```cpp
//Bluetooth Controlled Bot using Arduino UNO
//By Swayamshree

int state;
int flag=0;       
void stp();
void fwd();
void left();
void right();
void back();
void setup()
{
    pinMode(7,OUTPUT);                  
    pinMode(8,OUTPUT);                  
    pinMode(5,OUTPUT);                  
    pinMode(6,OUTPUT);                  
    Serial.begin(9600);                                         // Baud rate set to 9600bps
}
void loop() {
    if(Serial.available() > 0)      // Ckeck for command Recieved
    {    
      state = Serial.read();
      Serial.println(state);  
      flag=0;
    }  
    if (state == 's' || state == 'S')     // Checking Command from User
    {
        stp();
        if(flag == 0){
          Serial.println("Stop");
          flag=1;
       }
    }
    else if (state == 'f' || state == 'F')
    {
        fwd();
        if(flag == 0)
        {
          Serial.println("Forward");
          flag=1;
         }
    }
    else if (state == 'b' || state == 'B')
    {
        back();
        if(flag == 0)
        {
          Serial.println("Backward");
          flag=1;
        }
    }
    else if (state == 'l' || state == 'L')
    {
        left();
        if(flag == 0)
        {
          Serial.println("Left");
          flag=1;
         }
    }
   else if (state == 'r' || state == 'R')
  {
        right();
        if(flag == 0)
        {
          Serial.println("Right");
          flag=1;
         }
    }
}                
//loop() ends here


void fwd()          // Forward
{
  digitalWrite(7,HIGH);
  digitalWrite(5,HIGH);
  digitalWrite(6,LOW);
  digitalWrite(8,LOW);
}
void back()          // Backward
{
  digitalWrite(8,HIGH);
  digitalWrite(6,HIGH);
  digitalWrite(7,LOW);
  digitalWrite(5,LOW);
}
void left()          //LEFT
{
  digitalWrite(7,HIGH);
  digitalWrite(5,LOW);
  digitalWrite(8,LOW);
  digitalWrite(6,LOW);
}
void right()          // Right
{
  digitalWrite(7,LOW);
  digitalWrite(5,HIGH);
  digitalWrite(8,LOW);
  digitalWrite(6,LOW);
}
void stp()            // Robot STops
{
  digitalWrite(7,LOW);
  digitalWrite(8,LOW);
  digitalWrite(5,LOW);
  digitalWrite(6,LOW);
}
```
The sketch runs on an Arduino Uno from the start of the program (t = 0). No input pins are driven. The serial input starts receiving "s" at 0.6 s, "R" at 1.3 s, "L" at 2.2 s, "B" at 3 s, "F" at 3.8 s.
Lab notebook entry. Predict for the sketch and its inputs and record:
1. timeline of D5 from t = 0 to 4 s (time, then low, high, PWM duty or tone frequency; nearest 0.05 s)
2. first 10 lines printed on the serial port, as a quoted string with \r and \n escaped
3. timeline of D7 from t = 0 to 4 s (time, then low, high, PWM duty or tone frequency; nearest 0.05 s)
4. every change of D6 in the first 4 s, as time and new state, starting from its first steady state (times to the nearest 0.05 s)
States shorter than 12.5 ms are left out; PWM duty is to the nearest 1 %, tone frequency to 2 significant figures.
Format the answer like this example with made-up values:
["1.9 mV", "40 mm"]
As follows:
["0 s low; 1.3 s high; 2.2 s low; 3.8 s high", "\"115\\r\\nStop\\r\\n82\\r\\nRight\\r\\n76\\r\\nLeft\\r\\n66\\r\\nBackward\\r\\n70\\r\\nForward\\r\\n\"", "0 s low; 2.2 s high; 3 s low; 3.8 s high", "0 s low; 3 s high; 3.8 s low"]
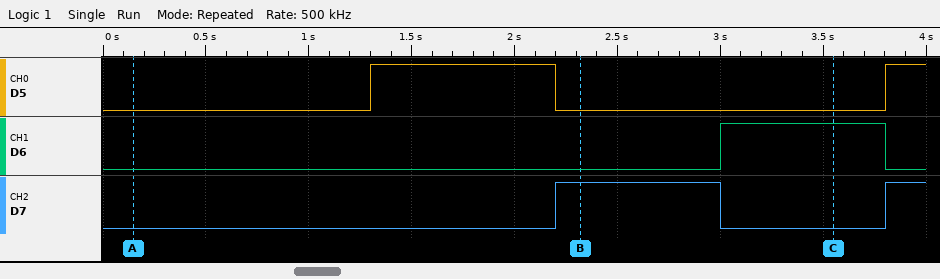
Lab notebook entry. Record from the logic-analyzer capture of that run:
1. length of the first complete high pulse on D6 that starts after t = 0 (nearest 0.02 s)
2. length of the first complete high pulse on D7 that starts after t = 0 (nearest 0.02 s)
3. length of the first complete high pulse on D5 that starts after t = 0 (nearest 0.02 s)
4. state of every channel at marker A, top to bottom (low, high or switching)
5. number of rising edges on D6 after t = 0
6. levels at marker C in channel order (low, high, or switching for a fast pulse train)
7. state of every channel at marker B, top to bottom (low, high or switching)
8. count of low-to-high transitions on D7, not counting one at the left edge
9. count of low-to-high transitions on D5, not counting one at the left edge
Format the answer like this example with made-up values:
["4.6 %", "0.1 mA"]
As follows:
["0.80 s", "0.80 s", "0.90 s", "D5 low, D6 low, D7 low", "1", "D5 low, D6 high, D7 low", "D5 low, D6 low, D7 high", "2", "2"]
